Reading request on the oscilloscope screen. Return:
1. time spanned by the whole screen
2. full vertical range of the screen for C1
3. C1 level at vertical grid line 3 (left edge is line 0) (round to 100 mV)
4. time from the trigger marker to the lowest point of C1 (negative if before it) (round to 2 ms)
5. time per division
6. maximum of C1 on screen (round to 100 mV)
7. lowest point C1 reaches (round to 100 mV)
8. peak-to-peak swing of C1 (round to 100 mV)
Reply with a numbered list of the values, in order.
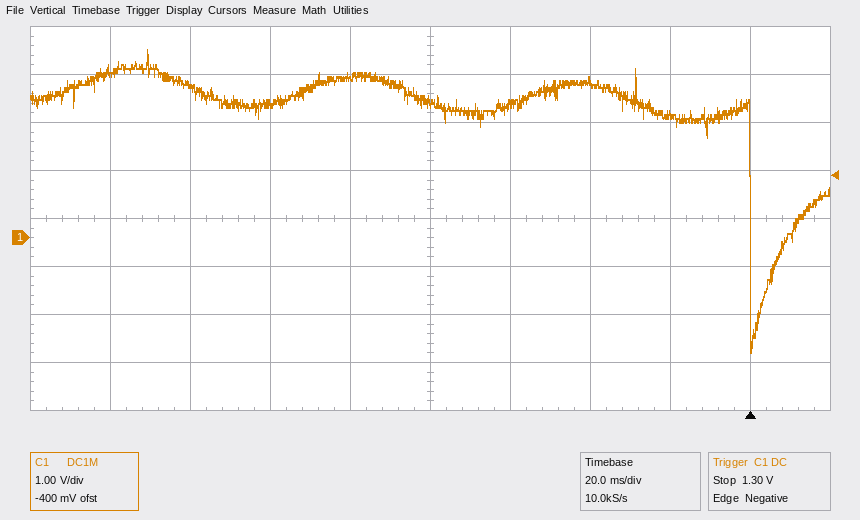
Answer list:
1. 200 ms
2. 8 V
3. 2.8 V
4. 0 ms
5. 20 ms
6. 3.9 V
7. -2.4 V
8. 6.3 V
